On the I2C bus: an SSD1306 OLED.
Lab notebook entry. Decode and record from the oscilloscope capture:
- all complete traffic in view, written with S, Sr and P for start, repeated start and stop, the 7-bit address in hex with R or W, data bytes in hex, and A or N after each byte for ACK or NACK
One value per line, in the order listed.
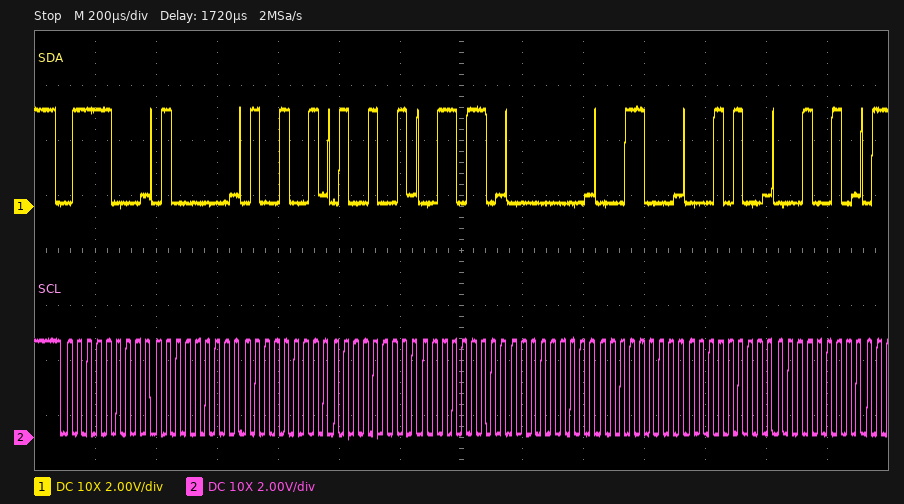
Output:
S 3CW A 40 A 49 A 49 A 36 A 00 A 18 A 14 A 12 A
